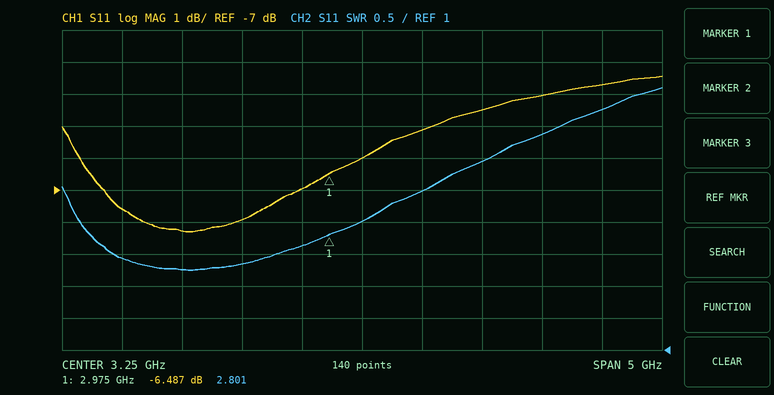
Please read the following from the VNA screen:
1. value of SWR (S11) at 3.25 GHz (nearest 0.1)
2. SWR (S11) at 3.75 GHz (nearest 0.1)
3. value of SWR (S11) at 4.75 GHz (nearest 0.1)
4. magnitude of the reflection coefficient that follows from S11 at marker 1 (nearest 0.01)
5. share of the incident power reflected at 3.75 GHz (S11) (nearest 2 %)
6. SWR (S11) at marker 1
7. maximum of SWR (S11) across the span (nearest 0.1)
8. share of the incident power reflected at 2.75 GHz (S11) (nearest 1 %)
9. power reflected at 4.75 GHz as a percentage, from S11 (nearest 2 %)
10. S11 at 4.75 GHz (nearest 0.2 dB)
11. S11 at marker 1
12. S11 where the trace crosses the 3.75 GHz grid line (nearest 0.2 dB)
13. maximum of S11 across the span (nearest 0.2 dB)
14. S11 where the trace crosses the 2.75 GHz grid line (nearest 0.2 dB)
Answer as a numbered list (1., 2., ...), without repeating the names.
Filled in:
1. 3.0
2. 3.5
3. 4.4
4. 0.47
5. 30 %
6. 2.801
7. 5.1
8. 20 %
9. 40 %
10. -4.0 dB
11. -6.487 dB
12. -5.2 dB
13. -3.4 dB
14. -7.0 dB
